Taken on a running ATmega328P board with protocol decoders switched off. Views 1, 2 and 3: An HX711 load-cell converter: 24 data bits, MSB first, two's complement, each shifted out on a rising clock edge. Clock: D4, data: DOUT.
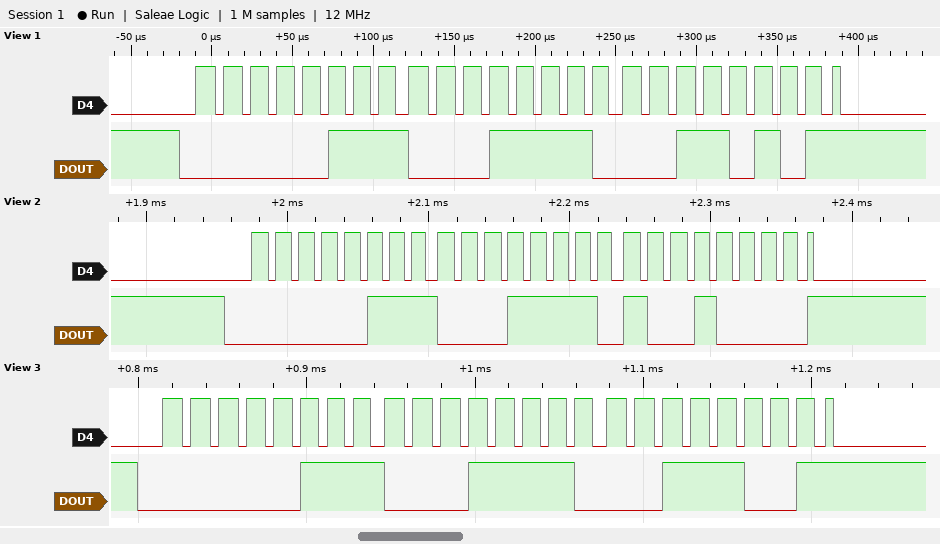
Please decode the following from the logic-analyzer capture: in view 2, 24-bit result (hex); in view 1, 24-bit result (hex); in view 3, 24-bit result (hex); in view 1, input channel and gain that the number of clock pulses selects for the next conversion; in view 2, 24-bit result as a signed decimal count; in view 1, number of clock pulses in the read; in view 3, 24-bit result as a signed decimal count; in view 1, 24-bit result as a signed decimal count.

0x071E90
0x071E35
0x071E39
channel A, gain 128
466576
25
466489
466485
